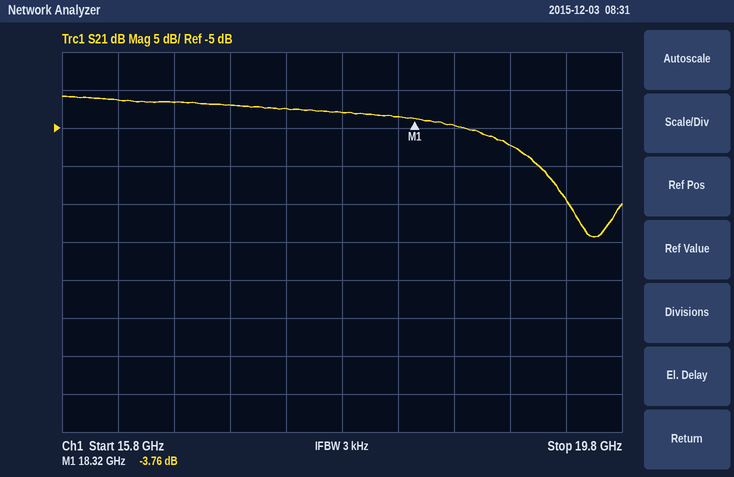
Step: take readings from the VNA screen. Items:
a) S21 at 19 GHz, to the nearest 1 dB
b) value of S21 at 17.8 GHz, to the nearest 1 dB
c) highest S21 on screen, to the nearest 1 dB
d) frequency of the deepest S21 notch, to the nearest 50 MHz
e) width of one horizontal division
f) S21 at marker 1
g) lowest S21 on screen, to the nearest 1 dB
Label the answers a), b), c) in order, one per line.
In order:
a) -7 dB
b) -3 dB
c) -1 dB
d) 19.60 GHz
e) 400 MHz
f) -3.76 dB
g) -19 dB
